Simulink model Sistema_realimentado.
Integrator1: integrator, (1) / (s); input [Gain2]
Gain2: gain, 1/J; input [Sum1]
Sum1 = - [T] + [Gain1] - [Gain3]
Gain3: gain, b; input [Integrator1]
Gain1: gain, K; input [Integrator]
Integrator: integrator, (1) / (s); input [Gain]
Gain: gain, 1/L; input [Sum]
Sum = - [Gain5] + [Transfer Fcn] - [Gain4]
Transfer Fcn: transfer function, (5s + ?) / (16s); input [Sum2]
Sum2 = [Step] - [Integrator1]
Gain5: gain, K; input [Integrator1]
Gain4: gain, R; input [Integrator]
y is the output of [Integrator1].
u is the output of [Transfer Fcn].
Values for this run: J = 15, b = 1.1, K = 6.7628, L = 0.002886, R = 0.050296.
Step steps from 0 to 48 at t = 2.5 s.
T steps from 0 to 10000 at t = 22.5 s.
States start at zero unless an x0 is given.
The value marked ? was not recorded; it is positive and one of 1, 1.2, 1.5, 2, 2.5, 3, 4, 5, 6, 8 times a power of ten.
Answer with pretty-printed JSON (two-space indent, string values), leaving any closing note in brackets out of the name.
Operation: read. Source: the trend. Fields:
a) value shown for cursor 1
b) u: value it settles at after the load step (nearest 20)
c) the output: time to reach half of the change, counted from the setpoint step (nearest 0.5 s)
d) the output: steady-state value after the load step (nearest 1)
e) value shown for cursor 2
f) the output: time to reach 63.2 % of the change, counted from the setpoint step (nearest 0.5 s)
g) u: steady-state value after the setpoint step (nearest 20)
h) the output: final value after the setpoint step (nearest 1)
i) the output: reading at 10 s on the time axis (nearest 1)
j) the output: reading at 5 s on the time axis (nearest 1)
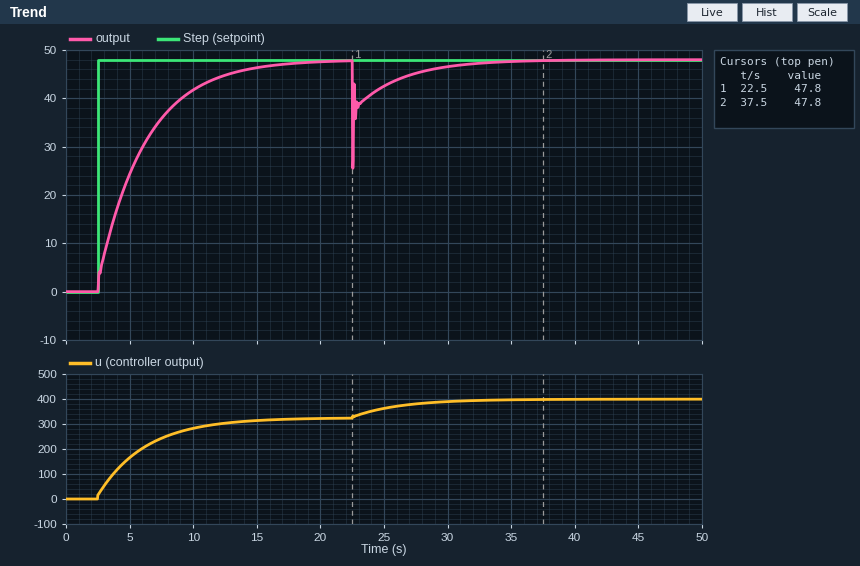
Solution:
{
  "value shown for cursor 1": "47.8",
  "u: value it settles at after the load step": "400",
  "the output: time to reach half of the change, counted from the setpoint step": "2.5 s",
  "the output: steady-state value after the load step": "48",
  "value shown for cursor 2": "47.8",
  "the output: time to reach 63.2 % of the change, counted from the setpoint step": "3.5 s",
  "u: steady-state value after the setpoint step": "320",
  "the output: final value after the setpoint step": "48",
  "the output: reading at 10 s on the time axis": "42",
  "the output: reading at 5 s on the time axis": "24"
}
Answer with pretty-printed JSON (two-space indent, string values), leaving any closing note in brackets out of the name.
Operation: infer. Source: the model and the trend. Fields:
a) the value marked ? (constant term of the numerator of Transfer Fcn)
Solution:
{
  "the value marked ?": "30"
}
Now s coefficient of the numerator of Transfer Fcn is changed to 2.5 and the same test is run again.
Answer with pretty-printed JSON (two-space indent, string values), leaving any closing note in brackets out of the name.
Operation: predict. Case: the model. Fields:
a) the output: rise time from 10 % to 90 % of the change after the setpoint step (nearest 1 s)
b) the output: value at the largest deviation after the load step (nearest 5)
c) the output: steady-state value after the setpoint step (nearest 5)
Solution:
{
  "the output: rise time from 10 % to 90 % of the change after the setpoint step": "8 s",
  "the output: value at the largest deviation after the load step": "25",
  "the output: steady-state value after the setpoint step": "50"
}
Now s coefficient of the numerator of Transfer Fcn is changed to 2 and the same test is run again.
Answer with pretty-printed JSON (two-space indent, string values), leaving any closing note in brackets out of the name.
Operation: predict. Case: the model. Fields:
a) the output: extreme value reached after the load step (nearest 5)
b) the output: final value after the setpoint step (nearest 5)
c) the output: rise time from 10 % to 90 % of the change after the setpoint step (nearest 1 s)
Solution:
{
  "the output: extreme value reached after the load step": "25",
  "the output: final value after the setpoint step": "50",
  "the output: rise time from 10 % to 90 % of the change after the setpoint step": "8 s"
}
